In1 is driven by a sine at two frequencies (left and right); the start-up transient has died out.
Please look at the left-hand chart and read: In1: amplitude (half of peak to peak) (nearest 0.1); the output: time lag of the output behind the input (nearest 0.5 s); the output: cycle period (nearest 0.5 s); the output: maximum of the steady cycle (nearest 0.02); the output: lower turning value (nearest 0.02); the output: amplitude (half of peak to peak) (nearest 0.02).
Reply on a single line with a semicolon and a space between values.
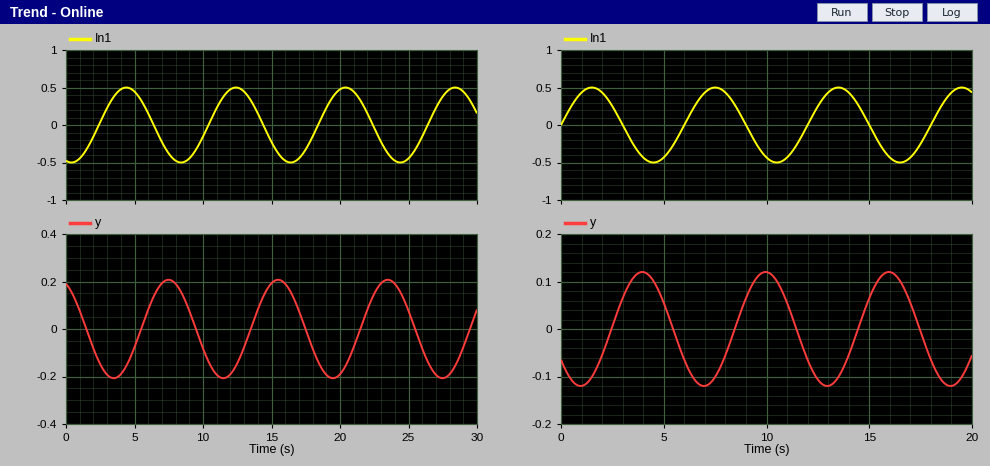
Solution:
0.5; 3.0 s; 8.0 s; 0.20; -0.20; 0.20
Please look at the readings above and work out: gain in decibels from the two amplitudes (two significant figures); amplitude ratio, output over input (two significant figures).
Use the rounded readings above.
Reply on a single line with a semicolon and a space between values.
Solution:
-8.0 dB; 0.40
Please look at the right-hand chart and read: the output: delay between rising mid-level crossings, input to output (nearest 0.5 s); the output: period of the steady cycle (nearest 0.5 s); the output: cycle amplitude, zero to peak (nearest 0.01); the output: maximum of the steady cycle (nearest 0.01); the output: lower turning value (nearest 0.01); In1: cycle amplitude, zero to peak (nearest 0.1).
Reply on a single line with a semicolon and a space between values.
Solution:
2.5 s; 6.0 s; 0.12; 0.12; -0.12; 0.5
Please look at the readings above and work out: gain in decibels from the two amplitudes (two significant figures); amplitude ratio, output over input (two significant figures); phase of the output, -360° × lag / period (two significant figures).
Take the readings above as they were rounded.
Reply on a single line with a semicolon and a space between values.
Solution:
-12 dB; 0.24; -150°
